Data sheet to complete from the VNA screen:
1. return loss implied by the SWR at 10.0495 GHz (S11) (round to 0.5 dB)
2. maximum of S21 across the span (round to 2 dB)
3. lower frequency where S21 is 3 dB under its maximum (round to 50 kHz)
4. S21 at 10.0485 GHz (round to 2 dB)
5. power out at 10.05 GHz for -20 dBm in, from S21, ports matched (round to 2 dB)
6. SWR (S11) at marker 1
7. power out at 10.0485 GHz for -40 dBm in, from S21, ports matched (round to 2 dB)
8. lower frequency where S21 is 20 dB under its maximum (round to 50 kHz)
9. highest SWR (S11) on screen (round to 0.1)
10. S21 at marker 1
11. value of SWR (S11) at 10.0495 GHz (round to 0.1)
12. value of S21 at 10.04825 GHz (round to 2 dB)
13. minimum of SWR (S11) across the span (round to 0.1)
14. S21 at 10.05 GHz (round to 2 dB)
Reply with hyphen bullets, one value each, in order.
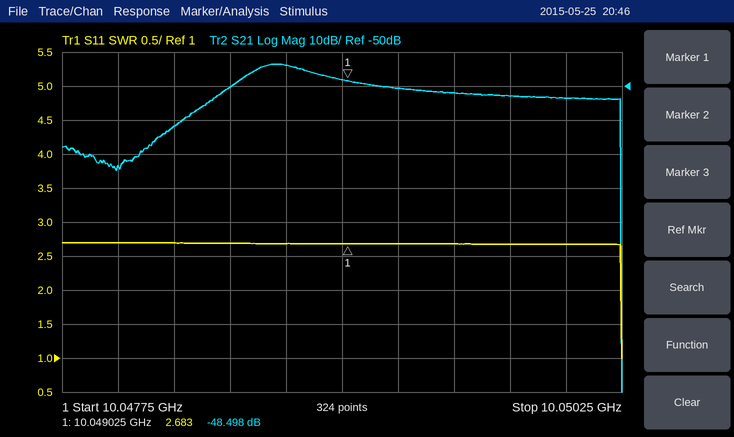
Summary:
- 7.0 dB
- -44 dB
- 10.04860 GHz
- -50 dB
- -74 dBm
- 2.683
- -90 dBm
- 10.04820 GHz
- 2.7
- -48.498 dB
- 2.7
- -62 dB
- 1.0
- -54 dB
